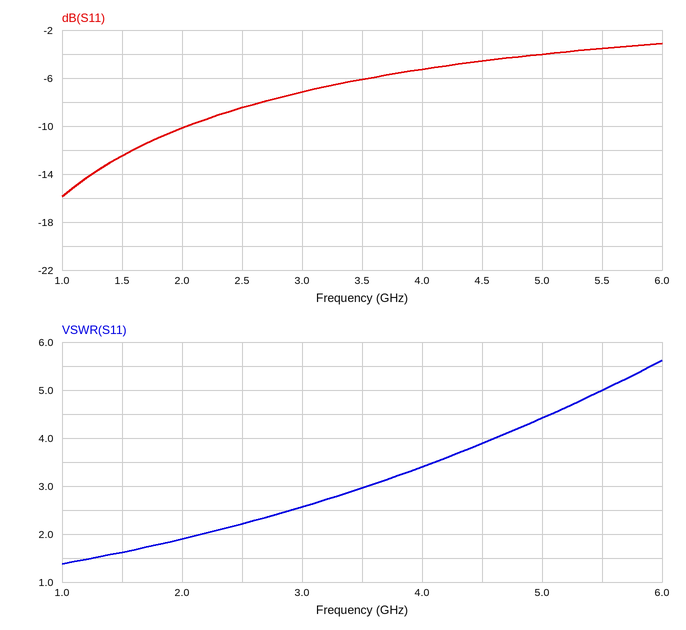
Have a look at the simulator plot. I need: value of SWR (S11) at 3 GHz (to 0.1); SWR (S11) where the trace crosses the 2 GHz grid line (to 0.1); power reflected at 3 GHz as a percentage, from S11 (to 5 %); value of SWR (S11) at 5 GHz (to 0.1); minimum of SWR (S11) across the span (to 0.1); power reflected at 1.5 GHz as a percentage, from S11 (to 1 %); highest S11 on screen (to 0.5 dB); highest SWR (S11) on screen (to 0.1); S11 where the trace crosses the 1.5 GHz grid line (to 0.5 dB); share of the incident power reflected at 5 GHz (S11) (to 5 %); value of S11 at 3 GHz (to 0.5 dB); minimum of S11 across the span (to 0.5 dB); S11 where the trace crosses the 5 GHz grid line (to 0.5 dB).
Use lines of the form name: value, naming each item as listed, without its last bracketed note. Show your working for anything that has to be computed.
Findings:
value of SWR (S11) at 3 GHz: 2.6
SWR (S11) where the trace crosses the 2 GHz grid line: 1.9
power reflected at 3 GHz as a percentage, from S11: 10^(-7/10) ≈ 20 %
value of SWR (S11) at 5 GHz: 4.4
minimum of SWR (S11) across the span: 1.4
power reflected at 1.5 GHz as a percentage, from S11: 10^(-12.5/10) ≈ 6 %
highest S11 on screen: -3.0 dB
highest SWR (S11) on screen: 5.6
S11 where the trace crosses the 1.5 GHz grid line: -12.5 dB
share of the incident power reflected at 5 GHz (S11): 10^(-4/10) ≈ 40 %
value of S11 at 3 GHz: -7.0 dB
minimum of S11 across the span: -16.0 dB
S11 where the trace crosses the 5 GHz grid line: -4.0 dB
